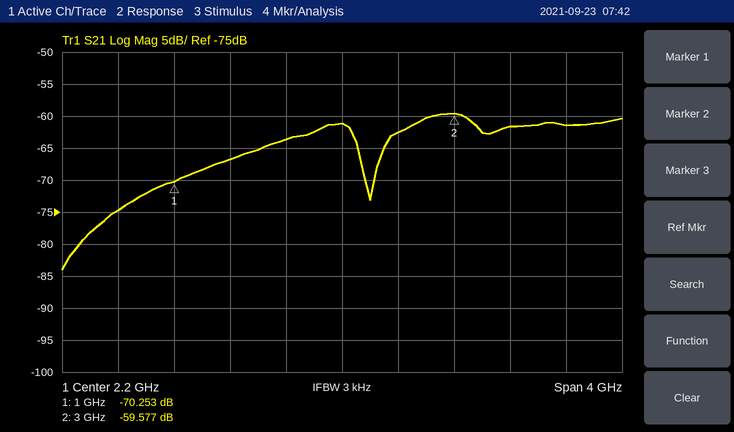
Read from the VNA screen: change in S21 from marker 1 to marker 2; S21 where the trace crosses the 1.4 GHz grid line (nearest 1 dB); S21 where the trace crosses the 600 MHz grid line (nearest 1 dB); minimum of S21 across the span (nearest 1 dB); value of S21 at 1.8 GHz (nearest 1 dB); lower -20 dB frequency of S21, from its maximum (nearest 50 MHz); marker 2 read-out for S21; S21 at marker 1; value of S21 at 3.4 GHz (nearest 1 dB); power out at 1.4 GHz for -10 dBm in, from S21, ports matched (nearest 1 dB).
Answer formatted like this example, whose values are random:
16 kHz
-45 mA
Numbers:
10.676 dB
-67 dB
-75 dB
-84 dB
-64 dB
350 MHz
-59.577 dB
-70.253 dB
-62 dB
-77 dBm
